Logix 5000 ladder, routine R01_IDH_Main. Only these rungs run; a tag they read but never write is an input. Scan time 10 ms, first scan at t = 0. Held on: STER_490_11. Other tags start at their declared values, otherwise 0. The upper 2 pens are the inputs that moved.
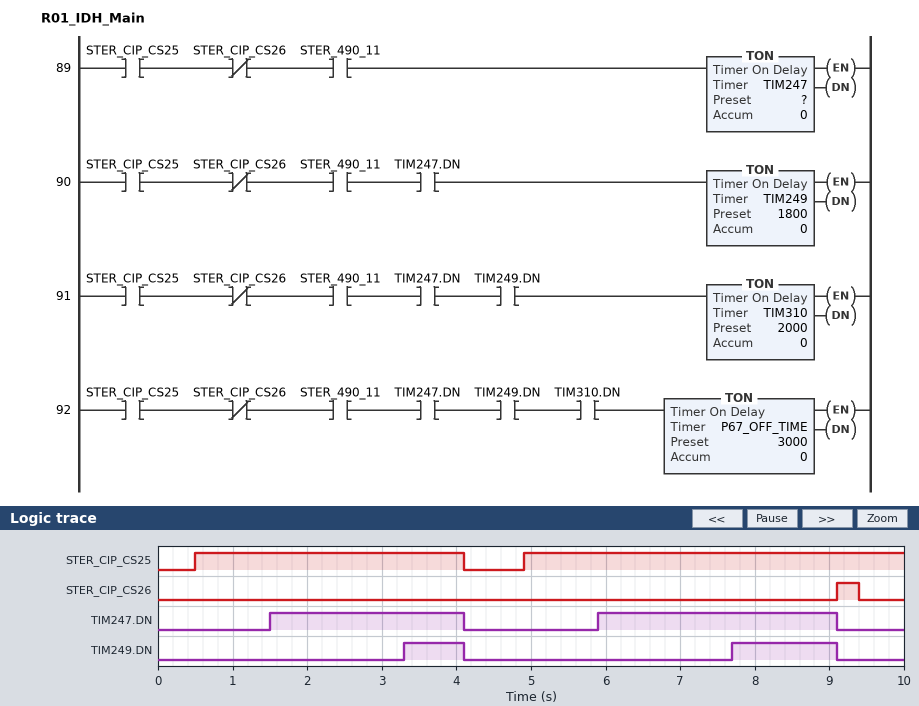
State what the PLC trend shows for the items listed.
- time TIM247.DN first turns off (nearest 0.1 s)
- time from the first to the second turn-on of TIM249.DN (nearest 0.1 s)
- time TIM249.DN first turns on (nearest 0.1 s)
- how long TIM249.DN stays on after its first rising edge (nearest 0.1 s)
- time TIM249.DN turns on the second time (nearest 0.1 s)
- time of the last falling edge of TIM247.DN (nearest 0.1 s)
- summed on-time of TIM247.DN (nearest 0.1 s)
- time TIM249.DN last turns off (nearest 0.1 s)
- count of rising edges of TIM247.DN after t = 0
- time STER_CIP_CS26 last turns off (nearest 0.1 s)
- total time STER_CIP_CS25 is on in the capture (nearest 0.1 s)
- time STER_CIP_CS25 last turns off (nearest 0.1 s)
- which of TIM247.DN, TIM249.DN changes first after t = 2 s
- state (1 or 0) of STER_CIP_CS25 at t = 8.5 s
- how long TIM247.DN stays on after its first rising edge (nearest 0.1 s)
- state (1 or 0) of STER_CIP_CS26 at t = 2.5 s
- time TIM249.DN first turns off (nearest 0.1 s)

4.1 s
4.4 s
3.3 s
0.8 s
7.7 s
9.1 s
5.8 s
9.1 s
2
9.4 s
8.7 s
4.1 s
TIM249.DN
1
2.6 s
0
4.1 s
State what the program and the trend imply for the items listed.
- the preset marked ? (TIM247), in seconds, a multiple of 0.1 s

1.0 s
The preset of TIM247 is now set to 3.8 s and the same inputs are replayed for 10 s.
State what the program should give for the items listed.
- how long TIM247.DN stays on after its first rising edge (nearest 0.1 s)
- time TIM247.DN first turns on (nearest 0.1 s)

0.4 s
8.7 s
